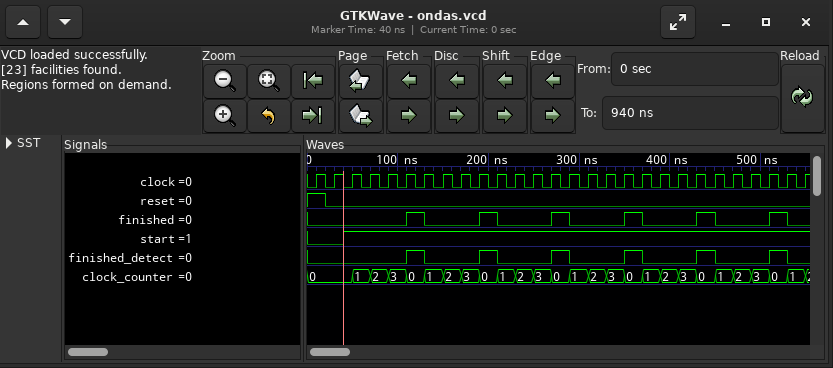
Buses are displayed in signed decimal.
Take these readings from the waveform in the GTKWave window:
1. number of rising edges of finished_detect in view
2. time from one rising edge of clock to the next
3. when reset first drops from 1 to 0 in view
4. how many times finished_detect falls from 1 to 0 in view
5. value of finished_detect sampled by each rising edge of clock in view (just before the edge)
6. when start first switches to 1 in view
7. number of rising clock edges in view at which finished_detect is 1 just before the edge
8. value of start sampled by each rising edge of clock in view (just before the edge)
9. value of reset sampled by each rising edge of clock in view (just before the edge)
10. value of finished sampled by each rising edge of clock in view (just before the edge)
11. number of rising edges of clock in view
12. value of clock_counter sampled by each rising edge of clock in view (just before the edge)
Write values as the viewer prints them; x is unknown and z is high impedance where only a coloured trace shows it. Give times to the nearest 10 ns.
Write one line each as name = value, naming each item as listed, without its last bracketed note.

number of rising edges of finished_detect in view = 6
time from one rising edge of clock to the next = 20 ns
when reset first drops from 1 to 0 in view = 20 ns
how many times finished_detect falls from 1 to 0 in view = 6
value of finished_detect sampled by each rising edge of clock in view = 0 0 0 0 0 0 1 0 0 0 1 0 0 0 1 0 0 0 1 0 0 0 1 0 0 0 1 0
when start first switches to 1 in view = 40 ns
number of rising clock edges in view at which finished_detect is 1 just before the edge = 6
value of start sampled by each rising edge of clock in view = 0 0 1 1 1 1 1 1 1 1 1 1 1 1 1 1 1 1 1 1 1 1 1 1 1 1 1 1
value of reset sampled by each rising edge of clock in view = 1 0 0 0 0 0 0 0 0 0 0 0 0 0 0 0 0 0 0 0 0 0 0 0 0 0 0 0
value of finished sampled by each rising edge of clock in view = 0 0 0 0 0 0 1 0 0 0 1 0 0 0 1 0 0 0 1 0 0 0 1 0 0 0 1 0
number of rising edges of clock in view = 28
value of clock_counter sampled by each rising edge of clock in view = 0, 0, 0, 1, 2, 3, 0, 1, 2, 3, 0, 1, 2, 3, 0, 1, 2, 3, 0, 1, 2, 3, 0, 1, 2, 3, 0, 1
